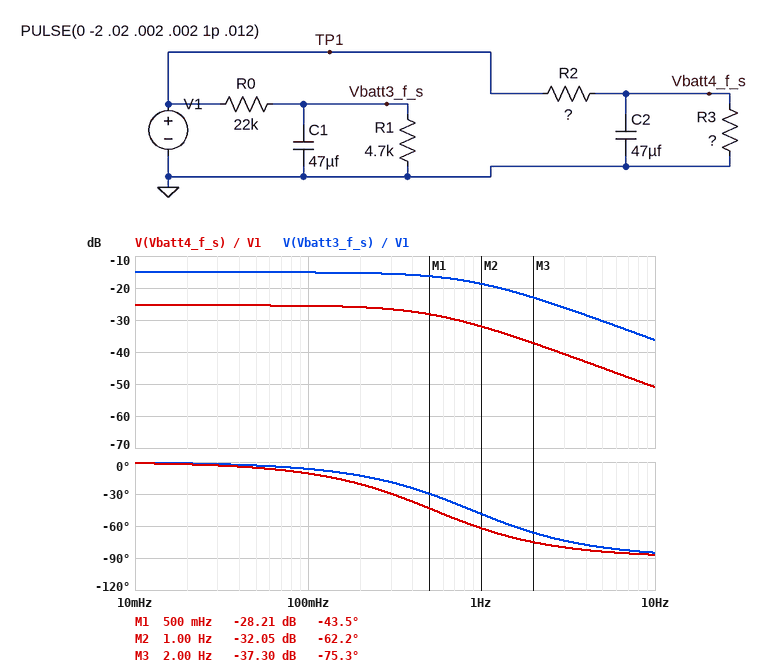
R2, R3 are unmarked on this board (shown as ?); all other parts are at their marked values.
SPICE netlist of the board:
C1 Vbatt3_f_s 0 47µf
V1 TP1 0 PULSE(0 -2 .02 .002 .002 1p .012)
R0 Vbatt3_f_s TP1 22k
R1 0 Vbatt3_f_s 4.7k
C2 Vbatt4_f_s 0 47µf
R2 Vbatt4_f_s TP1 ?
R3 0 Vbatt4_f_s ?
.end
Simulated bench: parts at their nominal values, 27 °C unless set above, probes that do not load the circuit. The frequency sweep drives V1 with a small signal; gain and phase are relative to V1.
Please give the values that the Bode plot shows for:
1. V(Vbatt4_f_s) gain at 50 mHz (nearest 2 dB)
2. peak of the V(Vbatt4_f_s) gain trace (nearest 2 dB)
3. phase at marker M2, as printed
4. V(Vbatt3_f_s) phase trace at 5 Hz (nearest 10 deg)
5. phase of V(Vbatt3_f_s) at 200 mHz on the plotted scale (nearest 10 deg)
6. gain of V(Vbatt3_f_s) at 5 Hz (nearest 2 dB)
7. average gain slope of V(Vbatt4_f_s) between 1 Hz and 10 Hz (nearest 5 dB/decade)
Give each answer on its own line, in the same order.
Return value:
-26 dB
-26 dB
-62.2 deg
-80 deg
-10 deg
-30 dB
-20 dB/decade
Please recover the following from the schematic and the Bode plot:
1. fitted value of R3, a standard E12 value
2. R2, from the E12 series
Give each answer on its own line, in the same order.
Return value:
6.8 kΩ
120 kΩ
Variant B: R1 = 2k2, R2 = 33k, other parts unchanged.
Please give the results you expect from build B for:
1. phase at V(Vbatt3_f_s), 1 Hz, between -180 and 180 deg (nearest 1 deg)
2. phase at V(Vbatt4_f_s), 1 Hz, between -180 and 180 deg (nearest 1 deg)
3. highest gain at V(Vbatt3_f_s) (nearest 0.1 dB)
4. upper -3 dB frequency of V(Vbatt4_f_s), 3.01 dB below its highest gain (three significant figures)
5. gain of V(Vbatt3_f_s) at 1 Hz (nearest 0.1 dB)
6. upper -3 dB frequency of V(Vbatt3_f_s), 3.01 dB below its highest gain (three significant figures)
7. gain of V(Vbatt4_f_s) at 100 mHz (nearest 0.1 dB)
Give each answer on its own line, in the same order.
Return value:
-31 deg
-59 deg
-20.8 dB
601 mHz
-22.1 dB
1.69 Hz
-15.5 dB
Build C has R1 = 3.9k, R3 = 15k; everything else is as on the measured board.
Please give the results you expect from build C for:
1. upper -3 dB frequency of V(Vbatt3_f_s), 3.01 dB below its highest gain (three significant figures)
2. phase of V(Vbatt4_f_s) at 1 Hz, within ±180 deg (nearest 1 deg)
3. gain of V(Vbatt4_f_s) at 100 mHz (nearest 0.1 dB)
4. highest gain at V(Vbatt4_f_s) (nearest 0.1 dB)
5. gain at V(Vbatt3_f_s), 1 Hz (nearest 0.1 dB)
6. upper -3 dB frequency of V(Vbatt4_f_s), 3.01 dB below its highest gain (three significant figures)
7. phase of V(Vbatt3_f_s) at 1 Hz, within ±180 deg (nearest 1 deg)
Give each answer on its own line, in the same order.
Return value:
1.02 Hz
-76 deg
-19.7 dB
-19.1 dB
-19.4 dB
254 mHz
-44 deg
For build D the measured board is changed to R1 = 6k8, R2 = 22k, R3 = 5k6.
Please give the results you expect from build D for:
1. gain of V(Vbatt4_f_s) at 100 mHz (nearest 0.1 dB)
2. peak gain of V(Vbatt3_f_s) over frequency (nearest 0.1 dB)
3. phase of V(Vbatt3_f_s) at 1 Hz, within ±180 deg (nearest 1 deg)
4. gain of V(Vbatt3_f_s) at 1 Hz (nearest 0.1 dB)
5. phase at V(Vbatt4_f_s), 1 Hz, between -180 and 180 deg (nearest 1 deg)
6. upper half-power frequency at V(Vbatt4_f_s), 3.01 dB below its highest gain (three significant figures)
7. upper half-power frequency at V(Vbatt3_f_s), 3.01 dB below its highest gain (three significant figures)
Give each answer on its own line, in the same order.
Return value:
-13.9 dB
-12.5 dB
-57 deg
-17.8 dB
-53 deg
759 mHz
652 mHz
